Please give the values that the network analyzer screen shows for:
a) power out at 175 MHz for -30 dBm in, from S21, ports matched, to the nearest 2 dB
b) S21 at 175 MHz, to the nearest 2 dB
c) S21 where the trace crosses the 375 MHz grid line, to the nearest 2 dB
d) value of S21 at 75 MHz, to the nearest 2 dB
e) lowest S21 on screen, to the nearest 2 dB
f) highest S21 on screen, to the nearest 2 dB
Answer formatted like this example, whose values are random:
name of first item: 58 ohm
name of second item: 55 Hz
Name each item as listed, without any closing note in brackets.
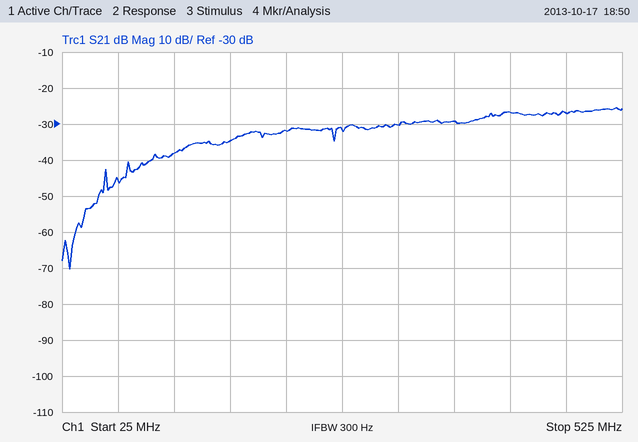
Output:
power out at 175 MHz for -30 dBm in, from S21, ports matched, to the nearest 2 dB: -64 dBm
S21 at 175 MHz, to the nearest 2 dB: -34 dB
S21 where the trace crosses the 375 MHz grid line, to the nearest 2 dB: -30 dB
value of S21 at 75 MHz, to the nearest 2 dB: -46 dB
lowest S21 on screen, to the nearest 2 dB: -70 dB
highest S21 on screen, to the nearest 2 dB: -26 dB
